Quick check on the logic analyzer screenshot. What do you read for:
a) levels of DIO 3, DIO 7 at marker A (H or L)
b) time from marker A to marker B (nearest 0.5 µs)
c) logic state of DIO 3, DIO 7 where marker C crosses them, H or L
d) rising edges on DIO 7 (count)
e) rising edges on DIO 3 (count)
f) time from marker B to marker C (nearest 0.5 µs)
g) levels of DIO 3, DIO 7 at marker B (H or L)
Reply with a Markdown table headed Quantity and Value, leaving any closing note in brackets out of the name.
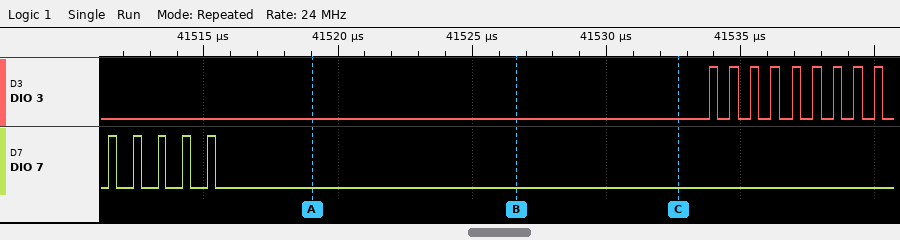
| Quantity | Value |
|---|---|
| levels of DIO 3, DIO 7 at marker A | DIO 3=L, DIO 7=L |
| time from marker A to marker B | 7.5 µs |
| logic state of DIO 3, DIO 7 where marker C crosses them, H or L | DIO 3=L, DIO 7=L |
| rising edges on DIO 7 | 5 |
| rising edges on DIO 3 | 9 |
| time from marker B to marker C | 6 µs |
| levels of DIO 3, DIO 7 at marker B | DIO 3=L, DIO 7=L |
